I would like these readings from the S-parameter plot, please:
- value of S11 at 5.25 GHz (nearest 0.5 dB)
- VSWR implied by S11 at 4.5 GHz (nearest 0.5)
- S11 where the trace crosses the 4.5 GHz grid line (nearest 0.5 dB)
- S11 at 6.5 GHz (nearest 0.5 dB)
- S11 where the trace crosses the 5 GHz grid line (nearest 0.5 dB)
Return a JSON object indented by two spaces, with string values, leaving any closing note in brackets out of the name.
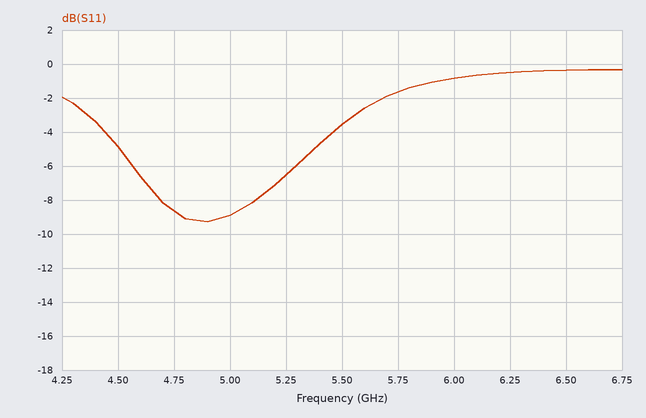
{
  "value of S11 at 5.25 GHz": "-6.5 dB",
  "VSWR implied by S11 at 4.5 GHz": "3.5",
  "S11 where the trace crosses the 4.5 GHz grid line": "-5.0 dB",
  "S11 at 6.5 GHz": "-0.5 dB",
  "S11 where the trace crosses the 5 GHz grid line": "-9.0 dB"
}
